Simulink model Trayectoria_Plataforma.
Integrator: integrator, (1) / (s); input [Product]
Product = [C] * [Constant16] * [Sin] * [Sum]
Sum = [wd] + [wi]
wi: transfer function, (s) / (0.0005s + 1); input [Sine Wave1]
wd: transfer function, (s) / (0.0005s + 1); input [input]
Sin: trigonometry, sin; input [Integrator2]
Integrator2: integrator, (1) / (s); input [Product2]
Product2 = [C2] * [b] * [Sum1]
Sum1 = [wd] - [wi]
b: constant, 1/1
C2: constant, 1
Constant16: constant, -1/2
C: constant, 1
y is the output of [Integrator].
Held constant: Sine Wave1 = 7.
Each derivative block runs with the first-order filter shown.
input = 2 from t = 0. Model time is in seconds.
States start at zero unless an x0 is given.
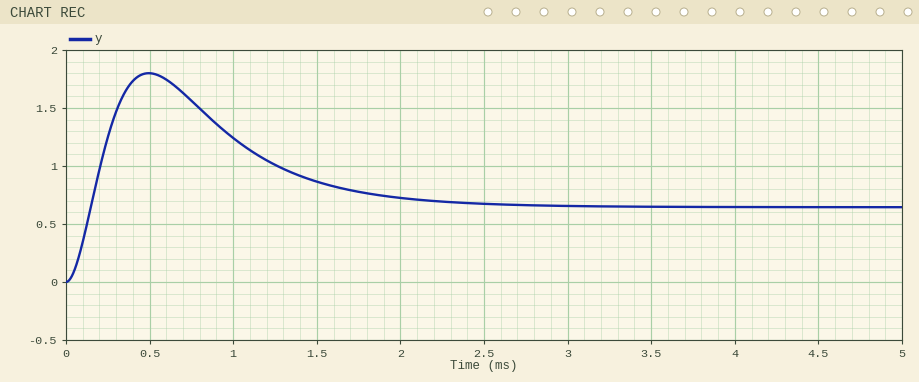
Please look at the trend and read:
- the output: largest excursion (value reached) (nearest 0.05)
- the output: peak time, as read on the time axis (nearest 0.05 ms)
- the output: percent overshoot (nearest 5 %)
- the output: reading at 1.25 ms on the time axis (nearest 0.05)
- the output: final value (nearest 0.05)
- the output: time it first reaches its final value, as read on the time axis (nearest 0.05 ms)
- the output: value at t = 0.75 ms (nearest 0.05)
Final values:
1.80
0.50 ms
180 %
1.00
0.65
0.15 ms
1.55
